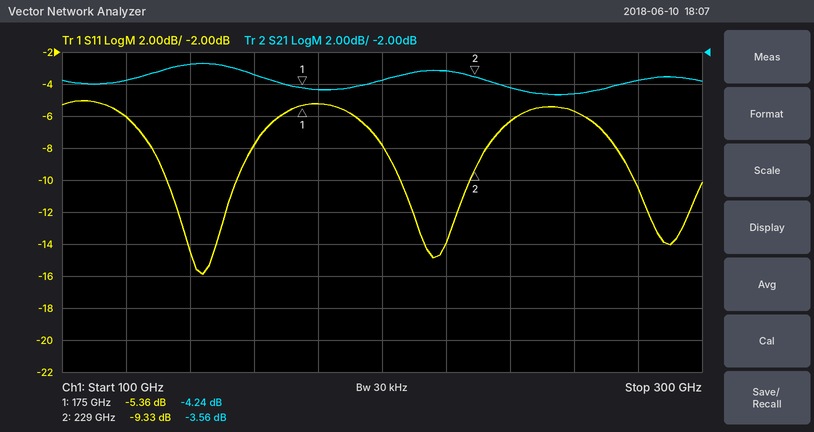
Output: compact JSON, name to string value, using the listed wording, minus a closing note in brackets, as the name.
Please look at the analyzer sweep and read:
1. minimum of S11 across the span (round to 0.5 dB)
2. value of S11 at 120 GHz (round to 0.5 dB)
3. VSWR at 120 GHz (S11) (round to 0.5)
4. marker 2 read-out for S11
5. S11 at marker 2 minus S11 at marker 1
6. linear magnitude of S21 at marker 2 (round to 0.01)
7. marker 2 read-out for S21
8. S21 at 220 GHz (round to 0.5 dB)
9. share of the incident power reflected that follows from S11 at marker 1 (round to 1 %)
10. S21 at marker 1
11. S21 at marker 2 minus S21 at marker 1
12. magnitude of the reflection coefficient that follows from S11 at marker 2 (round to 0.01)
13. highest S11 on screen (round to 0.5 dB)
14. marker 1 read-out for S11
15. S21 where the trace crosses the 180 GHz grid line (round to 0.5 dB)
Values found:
{"minimum of S11 across the span": "-16.0 dB", "value of S11 at 120 GHz": "-6.0 dB", "VSWR at 120 GHz (S11)": "3.0", "marker 2 read-out for S11": "-9.33 dB", "S11 at marker 2 minus S11 at marker 1": "-3.97 dB", "linear magnitude of S21 at marker 2": "0.66", "marker 2 read-out for S21": "-3.56 dB", "S21 at 220 GHz": "-3.0 dB", "share of the incident power reflected that follows from S11 at marker 1": "29 %", "S21 at marker 1": "-4.24 dB", "S21 at marker 2 minus S21 at marker 1": "0.68 dB", "magnitude of the reflection coefficient that follows from S11 at marker 2": "0.34", "highest S11 on screen": "-5.0 dB", "marker 1 read-out for S11": "-5.36 dB", "S21 where the trace crosses the 180 GHz grid line": "-4.5 dB"}
